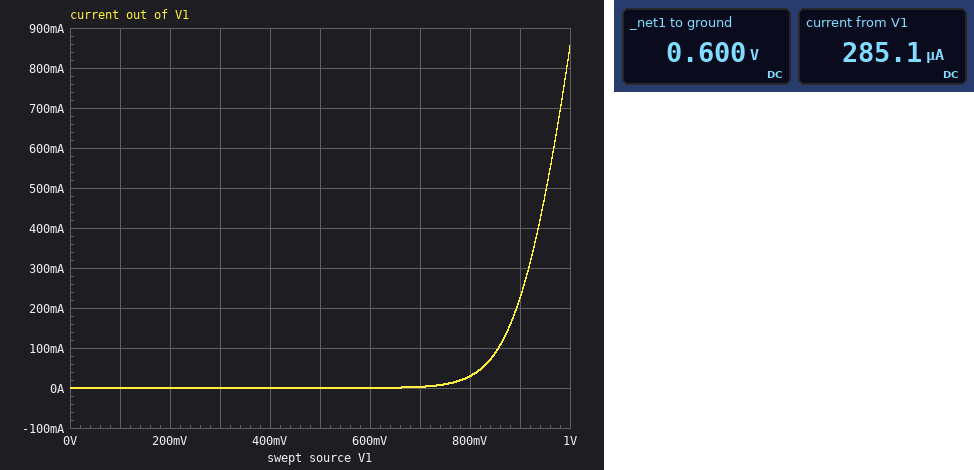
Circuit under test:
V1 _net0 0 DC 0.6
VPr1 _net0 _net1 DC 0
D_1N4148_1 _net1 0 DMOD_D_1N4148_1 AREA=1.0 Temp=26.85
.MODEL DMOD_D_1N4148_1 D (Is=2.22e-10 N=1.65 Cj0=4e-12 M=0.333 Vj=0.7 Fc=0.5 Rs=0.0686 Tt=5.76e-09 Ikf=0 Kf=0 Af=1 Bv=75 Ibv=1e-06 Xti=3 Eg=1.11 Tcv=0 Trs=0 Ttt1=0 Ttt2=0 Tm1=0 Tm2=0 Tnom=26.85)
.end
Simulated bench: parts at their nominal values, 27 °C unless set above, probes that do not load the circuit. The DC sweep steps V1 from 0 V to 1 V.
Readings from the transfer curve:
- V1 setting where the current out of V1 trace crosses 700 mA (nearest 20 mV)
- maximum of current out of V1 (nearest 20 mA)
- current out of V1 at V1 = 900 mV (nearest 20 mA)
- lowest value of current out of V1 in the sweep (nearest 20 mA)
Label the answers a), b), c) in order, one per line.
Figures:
a) 980 mV
b) 860 mA
c) 220 mA
d) 0 A
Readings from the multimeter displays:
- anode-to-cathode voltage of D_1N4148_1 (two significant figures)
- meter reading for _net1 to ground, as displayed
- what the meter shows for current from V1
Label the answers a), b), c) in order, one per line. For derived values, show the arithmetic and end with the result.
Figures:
a) 600 mV = 600 mV
b) 0.600 V
c) 285.1 µA
